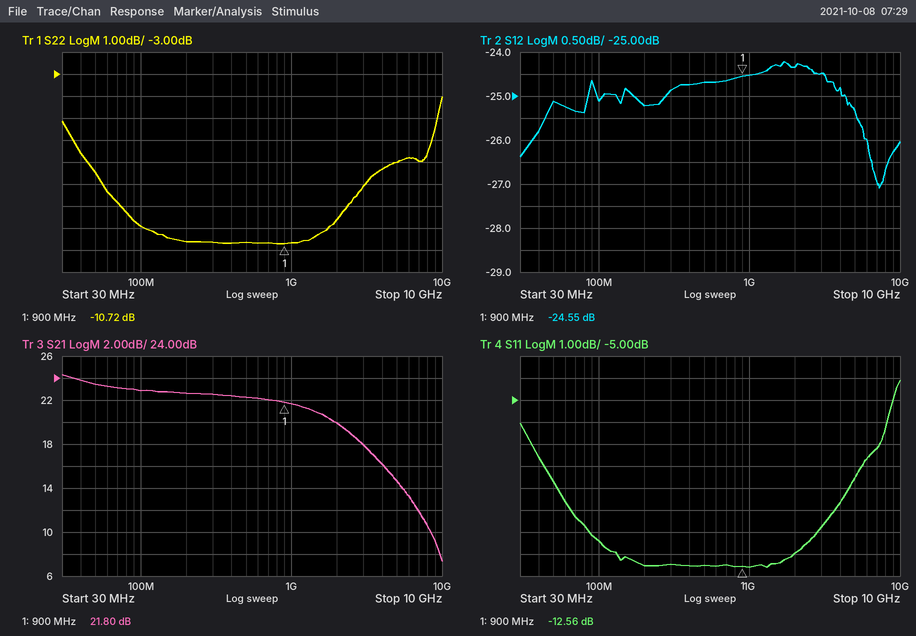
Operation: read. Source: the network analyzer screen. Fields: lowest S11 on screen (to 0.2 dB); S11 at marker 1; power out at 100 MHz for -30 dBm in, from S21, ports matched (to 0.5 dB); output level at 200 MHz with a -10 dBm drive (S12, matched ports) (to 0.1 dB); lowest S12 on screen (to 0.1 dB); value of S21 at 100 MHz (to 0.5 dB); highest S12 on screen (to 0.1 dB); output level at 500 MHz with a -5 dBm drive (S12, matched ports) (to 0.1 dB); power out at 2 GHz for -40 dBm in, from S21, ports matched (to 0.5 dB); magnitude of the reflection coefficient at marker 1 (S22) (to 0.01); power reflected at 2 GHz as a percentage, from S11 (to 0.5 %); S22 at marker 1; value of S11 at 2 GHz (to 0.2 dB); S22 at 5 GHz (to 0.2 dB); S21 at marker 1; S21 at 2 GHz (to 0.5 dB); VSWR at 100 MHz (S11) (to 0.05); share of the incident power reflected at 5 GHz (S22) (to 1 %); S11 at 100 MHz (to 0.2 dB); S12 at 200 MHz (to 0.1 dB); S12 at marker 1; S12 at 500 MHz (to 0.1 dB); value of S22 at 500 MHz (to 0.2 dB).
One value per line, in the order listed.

-12.6 dB
-12.56 dB
-7.0 dBm
-35.2 dBm
-27.1 dB
23.0 dB
-24.2 dB
-29.7 dBm
-20.0 dBm
0.29
6.5 %
-10.72 dB
-12.0 dB
-7.0 dB
21.80 dB
20.0 dB
1.75
20 %
-11.4 dB
-25.2 dB
-24.55 dB
-24.7 dB
-10.6 dB
